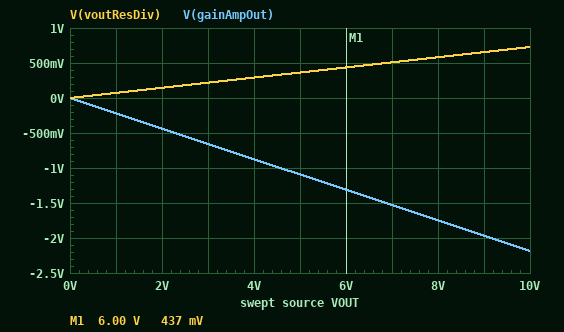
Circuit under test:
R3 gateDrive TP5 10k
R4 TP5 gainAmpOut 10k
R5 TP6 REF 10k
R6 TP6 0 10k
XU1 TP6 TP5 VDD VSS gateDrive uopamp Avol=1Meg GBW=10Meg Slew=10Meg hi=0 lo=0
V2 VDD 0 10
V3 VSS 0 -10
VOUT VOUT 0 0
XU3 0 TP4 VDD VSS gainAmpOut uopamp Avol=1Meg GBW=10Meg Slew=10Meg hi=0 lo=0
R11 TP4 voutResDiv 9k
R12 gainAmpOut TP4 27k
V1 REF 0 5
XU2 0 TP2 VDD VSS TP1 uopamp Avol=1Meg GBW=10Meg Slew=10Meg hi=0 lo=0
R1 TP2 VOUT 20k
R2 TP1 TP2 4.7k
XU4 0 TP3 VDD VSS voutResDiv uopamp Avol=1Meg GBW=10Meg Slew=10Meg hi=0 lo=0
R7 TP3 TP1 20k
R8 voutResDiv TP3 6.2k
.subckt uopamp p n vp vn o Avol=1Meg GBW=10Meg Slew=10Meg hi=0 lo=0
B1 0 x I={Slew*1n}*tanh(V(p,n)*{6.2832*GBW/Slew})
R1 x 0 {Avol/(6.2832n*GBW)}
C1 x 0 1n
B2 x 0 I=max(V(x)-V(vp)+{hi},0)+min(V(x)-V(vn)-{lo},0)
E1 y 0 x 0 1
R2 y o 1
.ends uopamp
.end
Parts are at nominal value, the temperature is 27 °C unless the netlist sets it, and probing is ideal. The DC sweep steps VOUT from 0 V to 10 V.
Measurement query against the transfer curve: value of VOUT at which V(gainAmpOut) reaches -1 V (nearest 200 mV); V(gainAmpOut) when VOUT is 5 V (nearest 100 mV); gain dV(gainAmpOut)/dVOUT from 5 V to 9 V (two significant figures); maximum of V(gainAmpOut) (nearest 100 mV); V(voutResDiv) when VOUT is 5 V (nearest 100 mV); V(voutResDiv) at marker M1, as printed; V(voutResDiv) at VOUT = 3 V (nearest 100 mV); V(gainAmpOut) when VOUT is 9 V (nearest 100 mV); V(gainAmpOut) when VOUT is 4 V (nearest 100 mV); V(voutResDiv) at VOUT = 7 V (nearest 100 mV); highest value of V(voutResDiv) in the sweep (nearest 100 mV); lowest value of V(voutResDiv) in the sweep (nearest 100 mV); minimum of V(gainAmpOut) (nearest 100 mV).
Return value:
4.6 V
-1.1 V
-0.22 V/V
0 V
400 mV
437 mV
200 mV
-2.0 V
-900 mV
500 mV
700 mV
0 V
-2.2 V
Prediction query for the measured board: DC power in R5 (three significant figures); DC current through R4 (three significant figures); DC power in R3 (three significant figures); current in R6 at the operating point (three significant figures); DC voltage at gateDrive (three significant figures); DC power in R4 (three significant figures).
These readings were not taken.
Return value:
625 µW
250 µA
625 µW
250 µA
5.00 V
625 µW
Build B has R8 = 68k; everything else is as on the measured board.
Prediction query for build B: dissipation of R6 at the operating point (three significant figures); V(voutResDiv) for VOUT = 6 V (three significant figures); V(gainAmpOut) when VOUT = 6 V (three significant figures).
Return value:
625 µW
4.79 V
-10.0 V
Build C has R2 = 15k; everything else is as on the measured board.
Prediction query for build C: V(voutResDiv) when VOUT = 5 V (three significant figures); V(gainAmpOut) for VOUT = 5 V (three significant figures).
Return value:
1.16 V
-3.49 V
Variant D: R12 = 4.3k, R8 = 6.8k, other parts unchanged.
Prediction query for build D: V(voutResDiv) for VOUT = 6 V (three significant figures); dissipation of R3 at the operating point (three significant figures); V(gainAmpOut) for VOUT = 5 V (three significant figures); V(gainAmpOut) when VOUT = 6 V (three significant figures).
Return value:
479 mV
625 µW
-191 mV
-229 mV
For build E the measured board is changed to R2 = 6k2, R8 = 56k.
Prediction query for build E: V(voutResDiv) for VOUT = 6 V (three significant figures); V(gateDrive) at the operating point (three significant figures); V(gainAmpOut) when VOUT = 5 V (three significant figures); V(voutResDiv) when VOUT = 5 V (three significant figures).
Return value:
5.21 V
5.00 V
-10.0 V
4.34 V
